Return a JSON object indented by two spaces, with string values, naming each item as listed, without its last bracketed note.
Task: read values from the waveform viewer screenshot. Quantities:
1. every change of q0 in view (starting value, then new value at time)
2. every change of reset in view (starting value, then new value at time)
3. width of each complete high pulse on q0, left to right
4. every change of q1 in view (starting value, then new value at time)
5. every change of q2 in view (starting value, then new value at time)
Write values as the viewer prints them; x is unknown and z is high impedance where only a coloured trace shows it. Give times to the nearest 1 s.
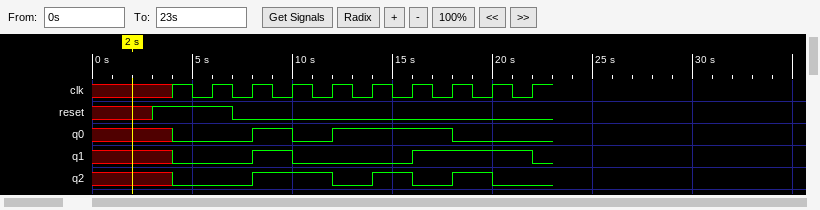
{
  "every change of q0 in view": "x, 0 at 4 s, 1 at 8 s, 0 at 10 s, 1 at 12 s, 0 at 18 s",
  "every change of reset in view": "x, 1 at 3 s, 0 at 7 s",
  "width of each complete high pulse on q0, left to right": "2 s, 6 s",
  "every change of q1 in view": "x, 0 at 4 s, 1 at 8 s, 0 at 10 s, 1 at 16 s, 0 at 22 s",
  "every change of q2 in view": "x, 0 at 4 s, 1 at 8 s, 0 at 12 s, 1 at 14 s, 0 at 16 s, 1 at 18 s, 0 at 20 s"
}
